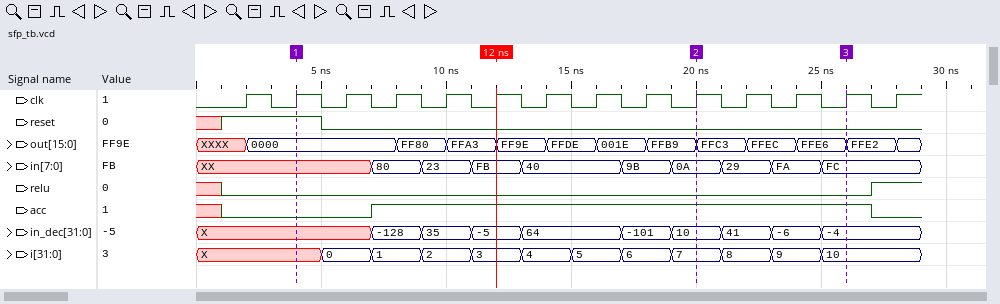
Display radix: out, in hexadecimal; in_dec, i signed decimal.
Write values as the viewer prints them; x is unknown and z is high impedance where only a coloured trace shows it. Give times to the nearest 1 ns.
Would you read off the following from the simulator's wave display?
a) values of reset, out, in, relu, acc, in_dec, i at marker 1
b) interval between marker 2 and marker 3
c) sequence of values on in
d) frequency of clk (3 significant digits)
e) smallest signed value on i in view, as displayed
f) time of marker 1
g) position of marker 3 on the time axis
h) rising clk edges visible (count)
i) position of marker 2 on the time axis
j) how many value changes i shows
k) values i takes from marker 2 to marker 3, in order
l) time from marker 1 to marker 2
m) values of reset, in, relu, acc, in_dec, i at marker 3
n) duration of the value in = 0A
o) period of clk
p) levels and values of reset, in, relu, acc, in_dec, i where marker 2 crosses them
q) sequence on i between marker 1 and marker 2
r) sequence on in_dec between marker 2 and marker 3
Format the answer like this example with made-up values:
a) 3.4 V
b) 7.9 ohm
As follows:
a) reset=1, out=0000, in=XX, relu=0, acc=0, in_dec=X, i=X
b) 6 ns
c) XX, 80, 23, FB, 40, 9B, 0A, 29, FA, FC
d) 500 MHz
e) 0
f) 4 ns
g) 26 ns
h) 14
i) 20 ns
j) 11
k) 7, 8, 9, 10
l) 16 ns
m) reset=0, in=FC, relu=0, acc=1, in_dec=-4, i=10
n) 2 ns
o) 2 ns
p) reset=0, in=0A, relu=0, acc=1, in_dec=10, i=7
q) X, 0, 1, 2, 3, 4, 5, 6, 7
r) 10, 41, -6, -4
